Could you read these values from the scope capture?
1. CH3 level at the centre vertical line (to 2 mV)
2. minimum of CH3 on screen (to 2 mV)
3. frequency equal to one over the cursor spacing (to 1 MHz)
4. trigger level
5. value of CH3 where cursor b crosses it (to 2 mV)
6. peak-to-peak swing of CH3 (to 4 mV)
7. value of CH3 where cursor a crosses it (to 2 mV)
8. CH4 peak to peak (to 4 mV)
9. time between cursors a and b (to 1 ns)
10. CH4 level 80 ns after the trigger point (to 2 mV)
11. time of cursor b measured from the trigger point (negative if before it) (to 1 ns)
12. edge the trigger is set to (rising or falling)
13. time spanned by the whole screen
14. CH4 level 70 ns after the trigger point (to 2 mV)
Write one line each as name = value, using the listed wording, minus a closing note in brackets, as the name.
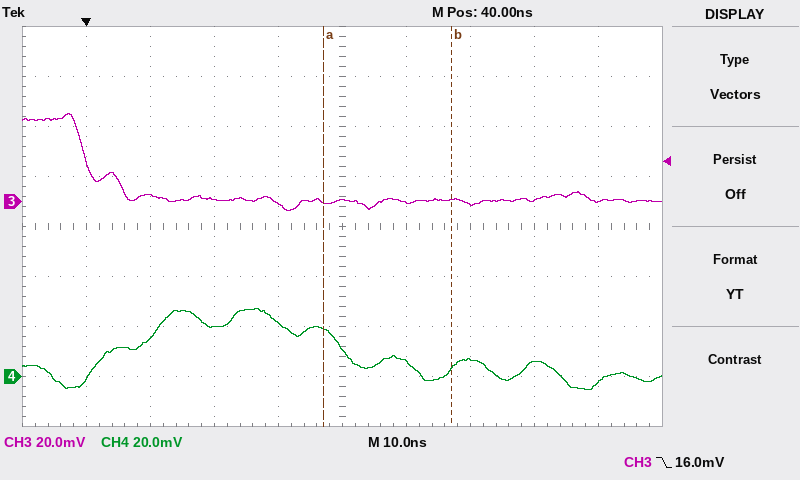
CH3 level at the centre vertical line = 0 mV
minimum of CH3 on screen = -4 mV
frequency equal to one over the cursor spacing = 50 MHz
trigger level = 16.0 mV
value of CH3 where cursor b crosses it = 0 mV
peak-to-peak swing of CH3 = 40 mV
value of CH3 where cursor a crosses it = 0 mV
CH4 peak to peak = 32 mV
time between cursors a and b = 20 ns
CH4 level 80 ns after the trigger point = -2 mV
time of cursor b measured from the trigger point (negative if before it) = +57 ns
edge the trigger is set to = falling
time spanned by the whole screen = 100 ns
CH4 level 70 ns after the trigger point = 6 mV
